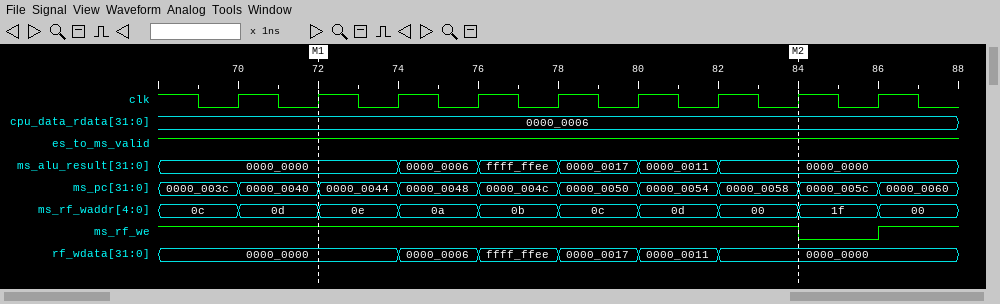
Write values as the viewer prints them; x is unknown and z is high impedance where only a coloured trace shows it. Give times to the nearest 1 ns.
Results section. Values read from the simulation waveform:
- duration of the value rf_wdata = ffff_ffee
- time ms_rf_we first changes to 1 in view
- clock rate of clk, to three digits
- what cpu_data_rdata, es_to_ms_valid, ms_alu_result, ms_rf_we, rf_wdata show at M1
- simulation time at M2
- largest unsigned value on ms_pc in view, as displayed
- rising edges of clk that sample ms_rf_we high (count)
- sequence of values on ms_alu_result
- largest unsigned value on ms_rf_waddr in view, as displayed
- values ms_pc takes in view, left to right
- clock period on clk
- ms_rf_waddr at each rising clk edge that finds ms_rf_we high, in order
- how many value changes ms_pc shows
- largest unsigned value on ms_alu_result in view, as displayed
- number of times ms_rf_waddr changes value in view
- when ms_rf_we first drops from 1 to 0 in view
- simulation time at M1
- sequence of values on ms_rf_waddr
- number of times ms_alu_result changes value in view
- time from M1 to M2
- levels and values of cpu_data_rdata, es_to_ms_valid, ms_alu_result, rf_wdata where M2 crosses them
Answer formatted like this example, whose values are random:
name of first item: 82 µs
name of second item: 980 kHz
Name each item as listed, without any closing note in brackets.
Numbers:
duration of the value rf_wdata = ffff_ffee: 2 ns
time ms_rf_we first changes to 1 in view: 86 ns
clock rate of clk, to three digits: 500 MHz
what cpu_data_rdata, es_to_ms_valid, ms_alu_result, ms_rf_we, rf_wdata show at M1: cpu_data_rdata=0000_0006, es_to_ms_valid=1, ms_alu_result=0000_0000, ms_rf_we=1, rf_wdata=0000_0000
simulation time at M2: 84 ns
largest unsigned value on ms_pc in view, as displayed: 0000_0060
rising edges of clk that sample ms_rf_we high: 8
sequence of values on ms_alu_result: 0000_0000, 0000_0006, ffff_ffee, 0000_0017, 0000_0011, 0000_0000
largest unsigned value on ms_rf_waddr in view, as displayed: 1f
values ms_pc takes in view, left to right: 0000_003c, 0000_0040, 0000_0044, 0000_0048, 0000_004c, 0000_0050, 0000_0054, 0000_0058, 0000_005c, 0000_0060
clock period on clk: 2 ns
ms_rf_waddr at each rising clk edge that finds ms_rf_we high, in order: 0c, 0d, 0e, 0a, 0b, 0c, 0d, 00
how many value changes ms_pc shows: 9
largest unsigned value on ms_alu_result in view, as displayed: ffff_ffee
number of times ms_rf_waddr changes value in view: 9
when ms_rf_we first drops from 1 to 0 in view: 84 ns
simulation time at M1: 72 ns
sequence of values on ms_rf_waddr: 0c, 0d, 0e, 0a, 0b, 0c, 0d, 00, 1f, 00
number of times ms_alu_result changes value in view: 5
time from M1 to M2: 12 ns
levels and values of cpu_data_rdata, es_to_ms_valid, ms_alu_result, rf_wdata where M2 crosses them: cpu_data_rdata=0000_0006, es_to_ms_valid=1, ms_alu_result=0000_0000, rf_wdata=0000_0000
